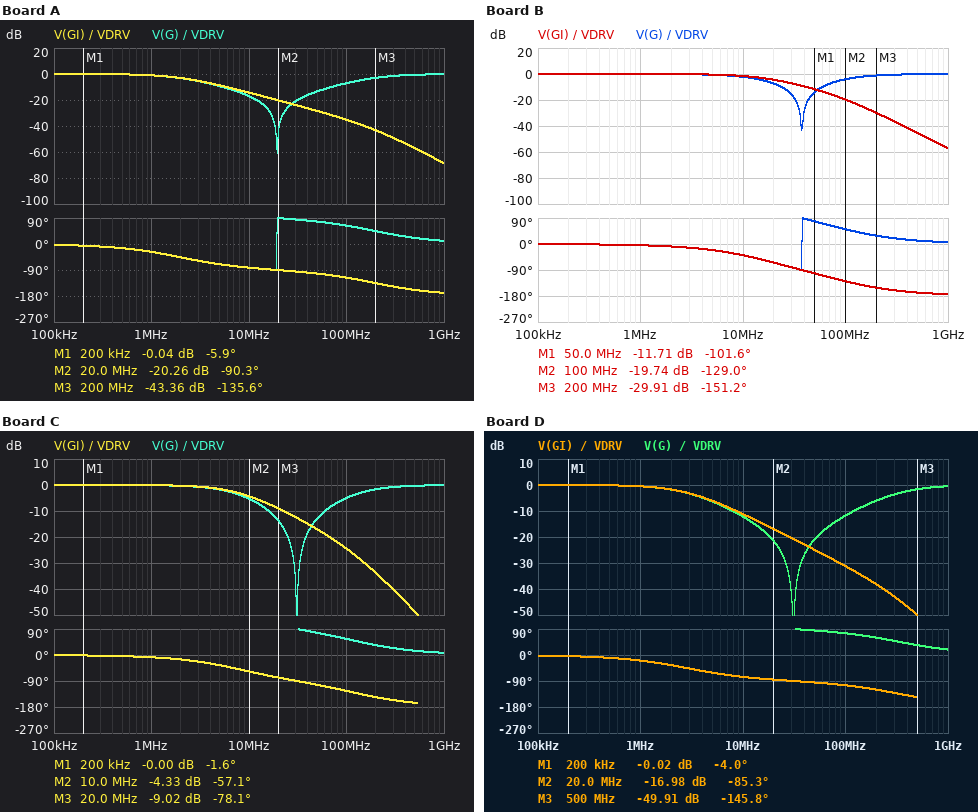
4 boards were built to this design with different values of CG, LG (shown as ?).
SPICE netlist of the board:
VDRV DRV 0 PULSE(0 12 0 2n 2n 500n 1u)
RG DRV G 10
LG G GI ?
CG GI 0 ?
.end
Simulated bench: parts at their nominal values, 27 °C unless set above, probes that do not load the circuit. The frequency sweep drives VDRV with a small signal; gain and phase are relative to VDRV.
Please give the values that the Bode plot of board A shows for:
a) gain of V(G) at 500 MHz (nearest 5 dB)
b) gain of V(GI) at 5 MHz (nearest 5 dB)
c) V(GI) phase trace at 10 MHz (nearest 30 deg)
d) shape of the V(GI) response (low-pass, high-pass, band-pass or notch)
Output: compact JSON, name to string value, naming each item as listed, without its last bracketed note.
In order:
{"gain of V(G) at 500 MHz": "0 dB", "gain of V(GI) at 5 MHz": "-10 dB", "V(GI) phase trace at 10 MHz": "-90 deg", "shape of the V(GI) response": "low-pass"}
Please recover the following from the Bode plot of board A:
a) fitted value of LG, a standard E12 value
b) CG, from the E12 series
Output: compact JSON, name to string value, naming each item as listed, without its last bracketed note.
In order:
{"fitted value of LG, a standard E12 value": "8.2 nH", "CG, from the E12 series": "8.2 nF"}
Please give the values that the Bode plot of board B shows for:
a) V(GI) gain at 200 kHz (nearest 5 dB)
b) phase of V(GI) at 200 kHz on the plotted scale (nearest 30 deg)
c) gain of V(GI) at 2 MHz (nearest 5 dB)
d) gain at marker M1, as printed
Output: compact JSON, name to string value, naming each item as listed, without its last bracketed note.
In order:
{"V(GI) gain at 200 kHz": "0 dB", "phase of V(GI) at 200 kHz on the plotted scale": "0 deg", "gain of V(GI) at 2 MHz": "0 dB", "gain at marker M1, as printed": "-11.71 dB"}
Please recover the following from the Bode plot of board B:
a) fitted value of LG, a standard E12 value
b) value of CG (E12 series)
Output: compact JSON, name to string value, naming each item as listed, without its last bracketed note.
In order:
{"fitted value of LG, a standard E12 value": "15 nH", "value of CG": "1.2 nF"}
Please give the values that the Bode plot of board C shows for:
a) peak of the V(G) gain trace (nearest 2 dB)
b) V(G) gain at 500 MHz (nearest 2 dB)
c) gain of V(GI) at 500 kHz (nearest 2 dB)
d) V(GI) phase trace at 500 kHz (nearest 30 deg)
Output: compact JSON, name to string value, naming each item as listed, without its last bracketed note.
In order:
{"peak of the V(G) gain trace": "0 dB", "V(G) gain at 500 MHz": "0 dB", "gain of V(GI) at 500 kHz": "0 dB", "V(GI) phase trace at 500 kHz": "0 deg"}
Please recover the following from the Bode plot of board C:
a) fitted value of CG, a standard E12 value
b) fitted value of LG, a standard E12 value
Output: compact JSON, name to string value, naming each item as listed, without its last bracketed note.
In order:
{"fitted value of CG, a standard E12 value": "2.2 nF", "fitted value of LG, a standard E12 value": "12 nH"}
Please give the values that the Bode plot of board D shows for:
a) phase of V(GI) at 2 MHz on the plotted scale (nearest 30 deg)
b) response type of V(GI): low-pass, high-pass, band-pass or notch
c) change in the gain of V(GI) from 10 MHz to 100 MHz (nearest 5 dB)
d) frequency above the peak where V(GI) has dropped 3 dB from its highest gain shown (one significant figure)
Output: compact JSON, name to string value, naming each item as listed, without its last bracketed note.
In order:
{"phase of V(GI) at 2 MHz on the plotted scale": "-30 deg", "response type of V(GI): low-pass, high-pass, band-pass or notch": "low-pass", "change in the gain of V(GI) from 10 MHz to 100 MHz": "-20 dB", "frequency above the peak where V(GI) has dropped 3 dB from its highest gain shown": "3 MHz"}
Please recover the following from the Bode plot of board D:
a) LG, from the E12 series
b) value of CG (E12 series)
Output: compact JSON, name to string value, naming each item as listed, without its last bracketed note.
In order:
{"LG, from the E12 series": "4.7 nH", "value of CG": "5.6 nF"}
